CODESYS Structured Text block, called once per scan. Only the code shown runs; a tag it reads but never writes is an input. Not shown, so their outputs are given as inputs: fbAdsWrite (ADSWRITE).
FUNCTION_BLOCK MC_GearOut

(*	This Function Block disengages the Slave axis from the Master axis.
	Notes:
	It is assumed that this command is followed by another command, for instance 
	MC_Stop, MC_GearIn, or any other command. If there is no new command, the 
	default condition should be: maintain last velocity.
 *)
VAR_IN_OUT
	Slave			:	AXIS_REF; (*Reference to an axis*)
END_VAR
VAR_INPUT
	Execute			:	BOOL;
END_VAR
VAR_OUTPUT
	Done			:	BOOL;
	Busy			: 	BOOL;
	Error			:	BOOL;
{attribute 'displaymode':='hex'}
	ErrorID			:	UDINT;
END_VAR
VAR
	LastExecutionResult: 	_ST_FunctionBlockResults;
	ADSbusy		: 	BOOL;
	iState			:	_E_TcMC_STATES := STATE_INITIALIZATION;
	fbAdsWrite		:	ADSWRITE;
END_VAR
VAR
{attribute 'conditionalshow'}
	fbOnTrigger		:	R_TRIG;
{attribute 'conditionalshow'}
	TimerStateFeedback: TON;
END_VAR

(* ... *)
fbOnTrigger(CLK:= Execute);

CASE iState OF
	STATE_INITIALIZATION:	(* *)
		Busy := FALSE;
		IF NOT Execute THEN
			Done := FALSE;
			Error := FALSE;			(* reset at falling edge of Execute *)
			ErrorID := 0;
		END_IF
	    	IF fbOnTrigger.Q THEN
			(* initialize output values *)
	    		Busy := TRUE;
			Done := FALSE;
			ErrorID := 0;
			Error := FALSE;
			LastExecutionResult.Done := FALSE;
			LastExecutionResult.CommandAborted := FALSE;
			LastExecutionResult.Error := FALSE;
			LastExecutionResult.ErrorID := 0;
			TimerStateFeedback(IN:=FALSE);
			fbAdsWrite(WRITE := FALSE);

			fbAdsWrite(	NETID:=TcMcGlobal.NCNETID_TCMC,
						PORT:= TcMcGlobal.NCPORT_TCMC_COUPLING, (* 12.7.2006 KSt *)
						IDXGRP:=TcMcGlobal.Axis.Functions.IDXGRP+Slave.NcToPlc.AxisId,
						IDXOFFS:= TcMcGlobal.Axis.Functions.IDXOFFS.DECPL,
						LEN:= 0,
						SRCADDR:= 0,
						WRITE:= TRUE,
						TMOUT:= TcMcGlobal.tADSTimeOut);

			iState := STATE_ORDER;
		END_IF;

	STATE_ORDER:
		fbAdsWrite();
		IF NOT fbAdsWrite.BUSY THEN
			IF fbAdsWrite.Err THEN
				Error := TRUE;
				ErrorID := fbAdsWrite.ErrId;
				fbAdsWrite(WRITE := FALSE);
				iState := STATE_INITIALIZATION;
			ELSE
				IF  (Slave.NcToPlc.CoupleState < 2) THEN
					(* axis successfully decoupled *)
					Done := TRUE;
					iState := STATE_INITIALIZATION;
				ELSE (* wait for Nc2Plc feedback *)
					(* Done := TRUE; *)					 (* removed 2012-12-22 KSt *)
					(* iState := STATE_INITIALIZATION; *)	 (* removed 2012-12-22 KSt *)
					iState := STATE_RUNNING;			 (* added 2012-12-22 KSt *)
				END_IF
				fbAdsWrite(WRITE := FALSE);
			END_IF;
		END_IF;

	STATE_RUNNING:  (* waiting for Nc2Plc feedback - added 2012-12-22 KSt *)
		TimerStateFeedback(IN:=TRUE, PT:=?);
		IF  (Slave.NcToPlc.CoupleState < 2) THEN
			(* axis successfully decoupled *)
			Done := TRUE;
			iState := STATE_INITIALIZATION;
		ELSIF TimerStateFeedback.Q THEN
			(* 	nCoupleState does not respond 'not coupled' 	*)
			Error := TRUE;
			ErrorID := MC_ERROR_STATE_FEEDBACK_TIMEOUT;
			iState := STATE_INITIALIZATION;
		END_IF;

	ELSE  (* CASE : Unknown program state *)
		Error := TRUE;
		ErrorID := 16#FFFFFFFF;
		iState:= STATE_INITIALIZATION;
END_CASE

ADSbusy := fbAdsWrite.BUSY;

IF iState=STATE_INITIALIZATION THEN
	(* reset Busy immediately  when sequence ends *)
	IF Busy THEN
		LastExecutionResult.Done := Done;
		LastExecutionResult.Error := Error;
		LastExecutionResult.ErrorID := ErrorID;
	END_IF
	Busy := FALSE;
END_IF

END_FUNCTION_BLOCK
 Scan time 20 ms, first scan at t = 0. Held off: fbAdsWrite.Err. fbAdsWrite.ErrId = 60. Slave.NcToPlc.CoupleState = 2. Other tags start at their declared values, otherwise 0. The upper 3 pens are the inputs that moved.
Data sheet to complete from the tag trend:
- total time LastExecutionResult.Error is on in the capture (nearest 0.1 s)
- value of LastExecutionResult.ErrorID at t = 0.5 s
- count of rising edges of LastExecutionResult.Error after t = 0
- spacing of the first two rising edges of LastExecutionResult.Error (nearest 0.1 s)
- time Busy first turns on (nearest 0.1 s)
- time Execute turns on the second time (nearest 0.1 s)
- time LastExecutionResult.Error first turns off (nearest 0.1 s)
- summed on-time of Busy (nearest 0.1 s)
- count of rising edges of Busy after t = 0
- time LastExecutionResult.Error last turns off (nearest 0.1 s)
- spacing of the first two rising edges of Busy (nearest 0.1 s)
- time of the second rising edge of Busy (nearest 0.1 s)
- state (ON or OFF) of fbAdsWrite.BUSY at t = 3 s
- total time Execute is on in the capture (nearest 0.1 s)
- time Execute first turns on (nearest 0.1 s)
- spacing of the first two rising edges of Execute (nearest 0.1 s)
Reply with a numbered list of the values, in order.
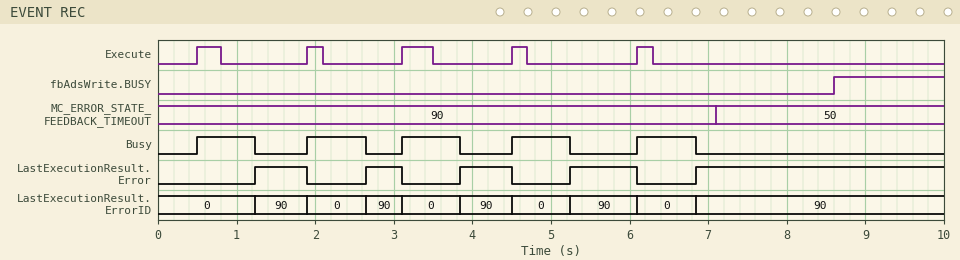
1. 5.8 s
2. 0
3. 5
4. 1.4 s
5. 0.5 s
6. 1.9 s
7. 1.9 s
8. 3.7 s
9. 5
10. 6.1 s
11. 1.4 s
12. 1.9 s
13. OFF
14. 1.3 s
15. 0.5 s
16. 1.4 s
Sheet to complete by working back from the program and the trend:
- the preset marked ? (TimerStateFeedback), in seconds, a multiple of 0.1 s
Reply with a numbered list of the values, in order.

1. 0.7 s
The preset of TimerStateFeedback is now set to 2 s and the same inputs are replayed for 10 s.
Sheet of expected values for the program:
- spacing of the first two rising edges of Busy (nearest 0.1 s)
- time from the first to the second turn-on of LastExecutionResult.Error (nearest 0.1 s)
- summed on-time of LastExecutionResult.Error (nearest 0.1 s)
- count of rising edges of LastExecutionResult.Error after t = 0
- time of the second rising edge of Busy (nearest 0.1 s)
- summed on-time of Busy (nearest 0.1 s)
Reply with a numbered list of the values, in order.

1. 2.6 s
2. 2.6 s
3. 3.4 s
4. 3
5. 3.1 s
6. 6.1 s
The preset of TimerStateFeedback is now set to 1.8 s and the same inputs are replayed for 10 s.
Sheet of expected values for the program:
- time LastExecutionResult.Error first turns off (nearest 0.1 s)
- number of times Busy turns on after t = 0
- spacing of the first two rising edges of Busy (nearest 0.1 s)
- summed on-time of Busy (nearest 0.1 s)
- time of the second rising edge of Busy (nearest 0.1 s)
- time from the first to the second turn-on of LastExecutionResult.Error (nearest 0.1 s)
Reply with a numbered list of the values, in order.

1. 3.1 s
2. 3
3. 2.6 s
4. 5.5 s
5. 3.1 s
6. 2.6 s
